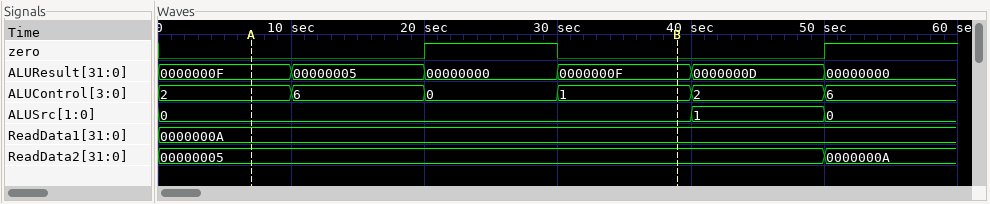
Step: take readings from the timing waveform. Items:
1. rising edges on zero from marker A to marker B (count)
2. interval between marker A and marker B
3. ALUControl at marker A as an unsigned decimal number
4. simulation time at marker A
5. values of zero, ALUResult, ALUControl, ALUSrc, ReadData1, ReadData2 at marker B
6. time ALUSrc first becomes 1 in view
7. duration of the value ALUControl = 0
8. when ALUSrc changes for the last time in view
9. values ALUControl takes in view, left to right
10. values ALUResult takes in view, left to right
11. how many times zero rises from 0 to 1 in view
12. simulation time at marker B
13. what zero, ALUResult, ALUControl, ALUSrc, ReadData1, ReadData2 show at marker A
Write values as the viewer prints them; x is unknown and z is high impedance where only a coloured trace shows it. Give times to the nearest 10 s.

1
30 s
2
10 s
zero=0, ALUResult=0000000F, ALUControl=1, ALUSrc=0, ReadData1=0000000A, ReadData2=00000005
40 s
10 s
50 s
2, 6, 0, 1, 2, 6
0000000F, 00000005, 00000000, 0000000F, 0000000D, 00000000
2
40 s
zero=0, ALUResult=0000000F, ALUControl=2, ALUSrc=0, ReadData1=0000000A, ReadData2=00000005
